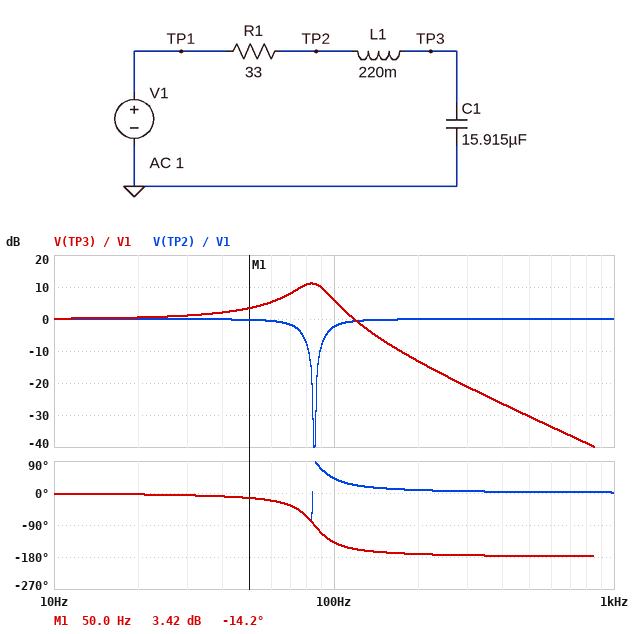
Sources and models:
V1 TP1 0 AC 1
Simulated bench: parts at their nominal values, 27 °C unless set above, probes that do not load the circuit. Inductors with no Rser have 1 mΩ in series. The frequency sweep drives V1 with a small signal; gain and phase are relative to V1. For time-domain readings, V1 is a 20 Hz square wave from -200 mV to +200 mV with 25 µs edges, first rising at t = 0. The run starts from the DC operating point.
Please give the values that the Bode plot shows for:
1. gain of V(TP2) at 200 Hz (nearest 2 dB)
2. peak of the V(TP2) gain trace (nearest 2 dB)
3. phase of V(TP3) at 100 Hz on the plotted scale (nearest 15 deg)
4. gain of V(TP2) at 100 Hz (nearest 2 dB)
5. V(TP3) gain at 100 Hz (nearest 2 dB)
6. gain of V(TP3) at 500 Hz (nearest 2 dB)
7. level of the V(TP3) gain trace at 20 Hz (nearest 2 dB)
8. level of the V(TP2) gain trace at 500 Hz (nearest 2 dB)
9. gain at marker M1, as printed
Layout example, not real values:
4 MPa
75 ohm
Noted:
0 dB
0 dB
-135 deg
-2 dB
6 dB
-30 dB
0 dB
0 dB
3.42 dB
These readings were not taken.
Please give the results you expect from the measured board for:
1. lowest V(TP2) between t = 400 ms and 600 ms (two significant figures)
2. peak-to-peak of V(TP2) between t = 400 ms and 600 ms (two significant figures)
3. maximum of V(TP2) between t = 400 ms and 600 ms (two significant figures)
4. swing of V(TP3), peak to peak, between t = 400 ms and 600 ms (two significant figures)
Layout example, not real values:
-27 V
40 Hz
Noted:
-250 mV
500 mV
250 mV
850 mV
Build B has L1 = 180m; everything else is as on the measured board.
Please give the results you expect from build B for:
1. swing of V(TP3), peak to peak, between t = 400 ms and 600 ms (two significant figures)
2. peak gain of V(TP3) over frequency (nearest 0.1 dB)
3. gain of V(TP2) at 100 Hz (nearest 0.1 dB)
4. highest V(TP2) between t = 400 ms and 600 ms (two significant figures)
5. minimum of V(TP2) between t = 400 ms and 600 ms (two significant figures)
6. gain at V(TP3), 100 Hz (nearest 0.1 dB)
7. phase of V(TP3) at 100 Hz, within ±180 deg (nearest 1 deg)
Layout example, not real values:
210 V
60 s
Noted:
900 mV
10.3 dB
-8.7 dB
260 mV
-260 mV
9.0 dB
-112 deg
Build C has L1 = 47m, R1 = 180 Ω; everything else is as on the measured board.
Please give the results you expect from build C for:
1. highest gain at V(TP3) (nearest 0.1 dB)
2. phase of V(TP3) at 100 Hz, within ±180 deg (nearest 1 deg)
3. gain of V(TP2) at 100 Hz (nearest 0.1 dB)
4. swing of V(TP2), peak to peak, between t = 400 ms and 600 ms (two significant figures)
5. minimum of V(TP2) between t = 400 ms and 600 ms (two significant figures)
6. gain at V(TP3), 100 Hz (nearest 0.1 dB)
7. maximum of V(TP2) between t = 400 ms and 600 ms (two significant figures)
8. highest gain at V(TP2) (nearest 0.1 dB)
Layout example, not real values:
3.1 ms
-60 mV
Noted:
0 dB
-69 deg
-8.8 dB
400 mV
-200 mV
-5.7 dB
200 mV
0 dB
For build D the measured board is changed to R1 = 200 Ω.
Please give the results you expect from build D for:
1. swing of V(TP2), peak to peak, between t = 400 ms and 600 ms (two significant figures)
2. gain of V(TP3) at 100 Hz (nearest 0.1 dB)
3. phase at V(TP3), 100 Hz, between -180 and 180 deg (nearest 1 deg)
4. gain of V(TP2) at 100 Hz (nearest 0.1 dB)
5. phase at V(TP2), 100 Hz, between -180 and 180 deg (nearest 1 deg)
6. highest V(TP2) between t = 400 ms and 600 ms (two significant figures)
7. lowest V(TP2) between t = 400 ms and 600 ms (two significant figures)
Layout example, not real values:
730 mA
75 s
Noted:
400 mV
-6.2 dB
-101 deg
-14.5 dB
79 deg
200 mV
-200 mV
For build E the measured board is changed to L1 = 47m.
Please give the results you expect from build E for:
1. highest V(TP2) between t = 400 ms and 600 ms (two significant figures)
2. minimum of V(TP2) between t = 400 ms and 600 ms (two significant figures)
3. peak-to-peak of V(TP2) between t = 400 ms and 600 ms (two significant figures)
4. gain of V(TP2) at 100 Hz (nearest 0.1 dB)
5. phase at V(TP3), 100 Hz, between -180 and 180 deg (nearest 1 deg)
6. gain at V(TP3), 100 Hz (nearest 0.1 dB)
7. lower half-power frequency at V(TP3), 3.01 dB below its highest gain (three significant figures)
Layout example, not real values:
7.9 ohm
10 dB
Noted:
260 mV
-260 mV
520 mV
-0.9 dB
-25 deg
2.2 dB
89.6 Hz
